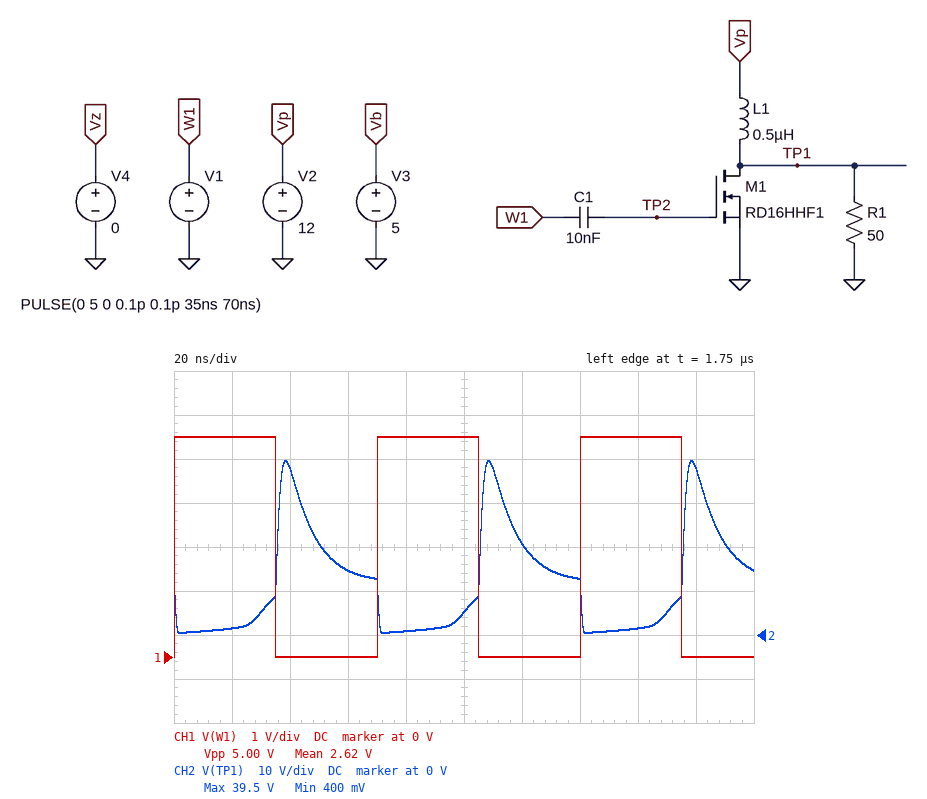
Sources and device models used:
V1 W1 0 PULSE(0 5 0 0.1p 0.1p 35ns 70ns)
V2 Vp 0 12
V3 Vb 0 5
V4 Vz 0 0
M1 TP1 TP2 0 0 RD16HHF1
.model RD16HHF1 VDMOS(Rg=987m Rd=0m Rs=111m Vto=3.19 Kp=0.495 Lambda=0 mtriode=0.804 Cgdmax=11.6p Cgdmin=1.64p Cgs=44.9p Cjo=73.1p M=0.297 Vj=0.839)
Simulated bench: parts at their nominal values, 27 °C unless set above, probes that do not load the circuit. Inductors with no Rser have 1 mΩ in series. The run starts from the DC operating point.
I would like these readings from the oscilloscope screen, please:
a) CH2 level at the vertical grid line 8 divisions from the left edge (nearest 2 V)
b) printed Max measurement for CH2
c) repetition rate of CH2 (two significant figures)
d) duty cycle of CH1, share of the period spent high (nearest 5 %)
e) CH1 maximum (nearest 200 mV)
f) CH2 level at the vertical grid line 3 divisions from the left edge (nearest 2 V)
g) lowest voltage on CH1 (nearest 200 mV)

2 V
39.5 V
14 MHz
50 %
5.0 V
14 V
0 V
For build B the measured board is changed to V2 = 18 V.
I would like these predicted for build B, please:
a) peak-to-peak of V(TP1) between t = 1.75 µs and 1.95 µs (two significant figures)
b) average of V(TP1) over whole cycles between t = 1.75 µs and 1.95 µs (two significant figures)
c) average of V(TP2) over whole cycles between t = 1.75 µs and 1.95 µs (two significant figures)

46 V
18 V
2.5 V
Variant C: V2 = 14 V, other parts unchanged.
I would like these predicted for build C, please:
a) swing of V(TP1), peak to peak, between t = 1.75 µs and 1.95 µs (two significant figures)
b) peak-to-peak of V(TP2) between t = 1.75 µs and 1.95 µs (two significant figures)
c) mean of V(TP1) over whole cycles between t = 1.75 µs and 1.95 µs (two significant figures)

42 V
5.0 V
14 V
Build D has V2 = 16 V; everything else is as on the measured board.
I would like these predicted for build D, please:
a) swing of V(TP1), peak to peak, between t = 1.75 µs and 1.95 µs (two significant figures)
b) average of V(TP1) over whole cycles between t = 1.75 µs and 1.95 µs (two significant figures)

44 V
16 V
